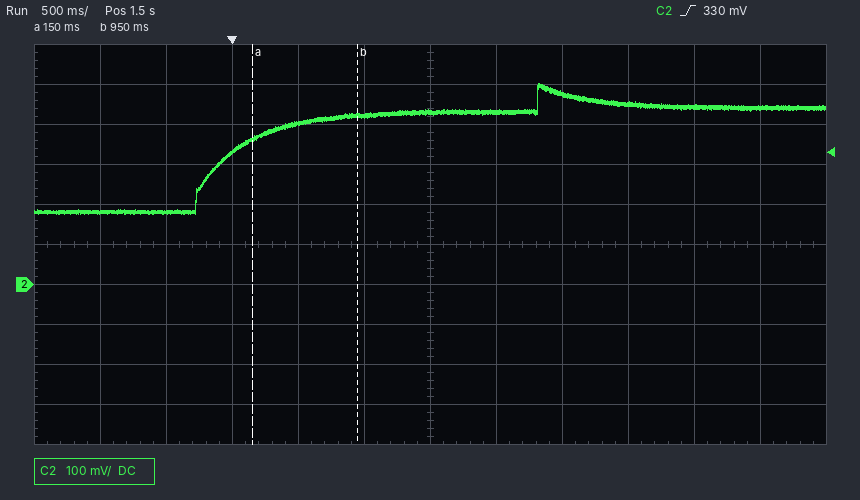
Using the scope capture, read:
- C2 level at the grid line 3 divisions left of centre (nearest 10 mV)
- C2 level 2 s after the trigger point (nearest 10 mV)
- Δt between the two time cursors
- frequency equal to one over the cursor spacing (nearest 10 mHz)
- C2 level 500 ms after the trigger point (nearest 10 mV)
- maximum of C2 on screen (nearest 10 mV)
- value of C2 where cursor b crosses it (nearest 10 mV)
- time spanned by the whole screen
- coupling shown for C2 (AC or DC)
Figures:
330 mV
430 mV
800 ms
1.25 Hz
400 mV
500 mV
420 mV
6 s
DC
